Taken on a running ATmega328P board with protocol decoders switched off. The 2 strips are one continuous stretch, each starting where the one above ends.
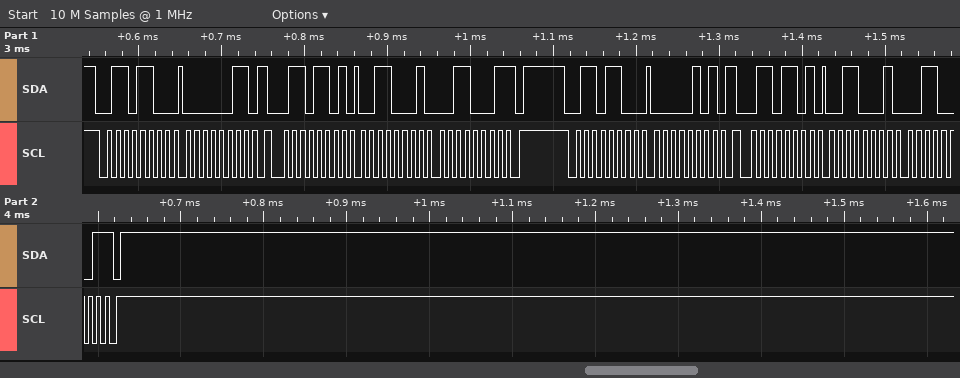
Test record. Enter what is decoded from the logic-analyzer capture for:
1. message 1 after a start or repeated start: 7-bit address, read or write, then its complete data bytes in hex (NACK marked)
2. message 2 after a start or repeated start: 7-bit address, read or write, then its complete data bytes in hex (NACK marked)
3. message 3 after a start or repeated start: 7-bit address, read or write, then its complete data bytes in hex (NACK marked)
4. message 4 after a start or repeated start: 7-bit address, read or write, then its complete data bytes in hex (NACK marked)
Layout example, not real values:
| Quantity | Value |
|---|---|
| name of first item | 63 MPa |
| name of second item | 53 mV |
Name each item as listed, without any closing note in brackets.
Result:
| Quantity | Value |
|---|---|
| message 1 after a start or repeated start: 7-bit address, read or write, then its complete data bytes in hex | 0x36 write: 03 |
| message 2 after a start or repeated start: 7-bit address, read or write, then its complete data bytes in hex | 0x36 read: 31 31 NACK |
| message 3 after a start or repeated start: 7-bit address, read or write, then its complete data bytes in hex | 0x36 write: 05 |
| message 4 after a start or repeated start: 7-bit address, read or write, then its complete data bytes in hex | 0x36 read: 31 31 NACK |
